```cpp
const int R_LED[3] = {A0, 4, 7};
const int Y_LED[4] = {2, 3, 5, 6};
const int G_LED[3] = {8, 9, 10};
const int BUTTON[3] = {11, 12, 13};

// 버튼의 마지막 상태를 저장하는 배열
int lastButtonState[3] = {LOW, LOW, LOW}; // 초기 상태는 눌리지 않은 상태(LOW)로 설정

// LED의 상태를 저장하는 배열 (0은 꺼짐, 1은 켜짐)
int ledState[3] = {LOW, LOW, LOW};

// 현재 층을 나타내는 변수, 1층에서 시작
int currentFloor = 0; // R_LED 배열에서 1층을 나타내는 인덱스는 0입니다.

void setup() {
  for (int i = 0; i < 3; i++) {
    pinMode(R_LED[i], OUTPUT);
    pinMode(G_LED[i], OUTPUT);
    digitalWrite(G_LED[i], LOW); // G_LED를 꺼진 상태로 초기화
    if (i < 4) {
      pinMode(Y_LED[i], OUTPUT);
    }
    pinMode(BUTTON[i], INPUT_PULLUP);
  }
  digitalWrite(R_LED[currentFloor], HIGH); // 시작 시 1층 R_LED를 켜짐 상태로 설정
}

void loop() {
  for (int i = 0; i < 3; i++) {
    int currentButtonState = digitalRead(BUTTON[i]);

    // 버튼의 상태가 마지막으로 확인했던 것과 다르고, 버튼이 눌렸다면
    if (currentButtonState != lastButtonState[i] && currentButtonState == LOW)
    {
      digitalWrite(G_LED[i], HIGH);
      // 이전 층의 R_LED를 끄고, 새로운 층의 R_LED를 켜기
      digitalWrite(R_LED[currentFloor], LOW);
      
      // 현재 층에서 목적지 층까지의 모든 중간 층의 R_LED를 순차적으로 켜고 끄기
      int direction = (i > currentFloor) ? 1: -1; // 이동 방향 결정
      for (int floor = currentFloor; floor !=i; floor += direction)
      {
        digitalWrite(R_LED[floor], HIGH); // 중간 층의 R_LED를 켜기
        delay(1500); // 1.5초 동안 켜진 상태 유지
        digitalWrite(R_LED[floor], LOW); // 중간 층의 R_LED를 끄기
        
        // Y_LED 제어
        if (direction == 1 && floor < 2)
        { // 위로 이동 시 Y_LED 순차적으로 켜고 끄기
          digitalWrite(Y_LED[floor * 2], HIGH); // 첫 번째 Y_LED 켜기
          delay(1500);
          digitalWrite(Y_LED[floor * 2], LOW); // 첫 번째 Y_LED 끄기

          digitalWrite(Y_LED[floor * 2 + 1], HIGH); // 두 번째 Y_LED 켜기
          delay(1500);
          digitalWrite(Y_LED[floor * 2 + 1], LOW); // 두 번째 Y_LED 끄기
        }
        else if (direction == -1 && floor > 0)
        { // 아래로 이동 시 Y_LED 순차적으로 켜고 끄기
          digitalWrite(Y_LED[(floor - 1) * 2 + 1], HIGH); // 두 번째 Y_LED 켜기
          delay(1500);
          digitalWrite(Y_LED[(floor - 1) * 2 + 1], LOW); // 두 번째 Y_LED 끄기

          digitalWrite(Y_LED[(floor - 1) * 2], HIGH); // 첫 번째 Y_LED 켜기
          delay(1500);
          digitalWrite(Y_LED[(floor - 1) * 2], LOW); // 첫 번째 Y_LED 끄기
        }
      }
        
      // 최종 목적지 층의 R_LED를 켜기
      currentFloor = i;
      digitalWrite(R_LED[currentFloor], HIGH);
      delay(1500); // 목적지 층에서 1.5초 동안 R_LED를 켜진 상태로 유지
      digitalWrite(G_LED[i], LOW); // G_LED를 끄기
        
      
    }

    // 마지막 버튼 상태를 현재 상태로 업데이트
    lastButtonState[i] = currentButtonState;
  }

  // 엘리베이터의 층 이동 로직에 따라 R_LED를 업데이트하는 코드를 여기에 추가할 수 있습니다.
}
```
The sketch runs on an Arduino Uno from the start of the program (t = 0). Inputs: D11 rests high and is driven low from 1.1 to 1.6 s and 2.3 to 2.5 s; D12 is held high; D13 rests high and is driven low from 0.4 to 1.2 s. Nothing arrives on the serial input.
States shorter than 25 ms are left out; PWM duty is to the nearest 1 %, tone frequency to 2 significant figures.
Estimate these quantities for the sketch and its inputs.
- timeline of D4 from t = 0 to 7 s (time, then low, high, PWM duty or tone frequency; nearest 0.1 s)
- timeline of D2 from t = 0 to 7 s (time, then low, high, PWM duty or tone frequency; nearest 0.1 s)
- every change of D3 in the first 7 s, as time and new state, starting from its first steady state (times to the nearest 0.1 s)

0 s low; 4.9 s high; 6.4 s low
0 s low; 1.9 s high; 3.4 s low
0 s low; 3.4 s high; 4.9 s low
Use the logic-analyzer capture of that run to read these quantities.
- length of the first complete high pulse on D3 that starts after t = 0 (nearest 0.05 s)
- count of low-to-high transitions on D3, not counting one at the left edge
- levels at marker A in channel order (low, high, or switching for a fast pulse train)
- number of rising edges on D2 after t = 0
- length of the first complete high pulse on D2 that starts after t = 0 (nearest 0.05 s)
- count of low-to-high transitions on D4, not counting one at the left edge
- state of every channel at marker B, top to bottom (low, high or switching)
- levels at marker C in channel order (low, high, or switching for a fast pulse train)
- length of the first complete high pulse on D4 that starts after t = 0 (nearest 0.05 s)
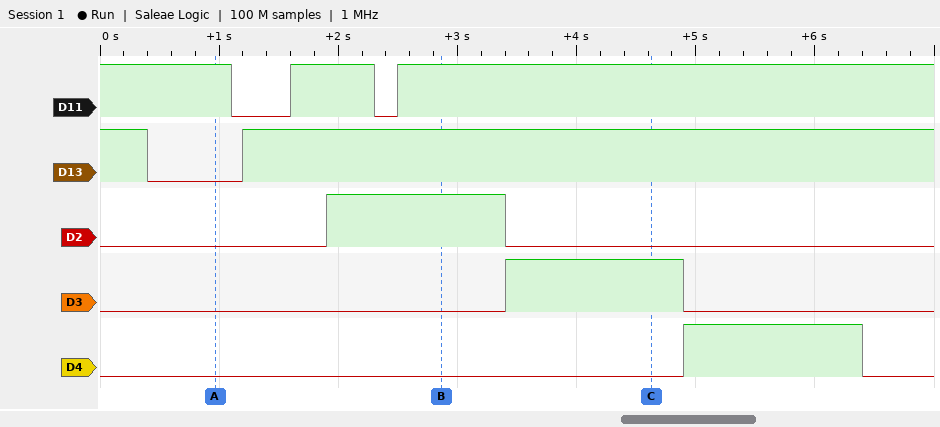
1.50 s
1
D11 high, D13 low, D2 low, D3 low, D4 low
1
1.50 s
1
D11 high, D13 high, D2 high, D3 low, D4 low
D11 high, D13 high, D2 low, D3 high, D4 low
1.50 s
